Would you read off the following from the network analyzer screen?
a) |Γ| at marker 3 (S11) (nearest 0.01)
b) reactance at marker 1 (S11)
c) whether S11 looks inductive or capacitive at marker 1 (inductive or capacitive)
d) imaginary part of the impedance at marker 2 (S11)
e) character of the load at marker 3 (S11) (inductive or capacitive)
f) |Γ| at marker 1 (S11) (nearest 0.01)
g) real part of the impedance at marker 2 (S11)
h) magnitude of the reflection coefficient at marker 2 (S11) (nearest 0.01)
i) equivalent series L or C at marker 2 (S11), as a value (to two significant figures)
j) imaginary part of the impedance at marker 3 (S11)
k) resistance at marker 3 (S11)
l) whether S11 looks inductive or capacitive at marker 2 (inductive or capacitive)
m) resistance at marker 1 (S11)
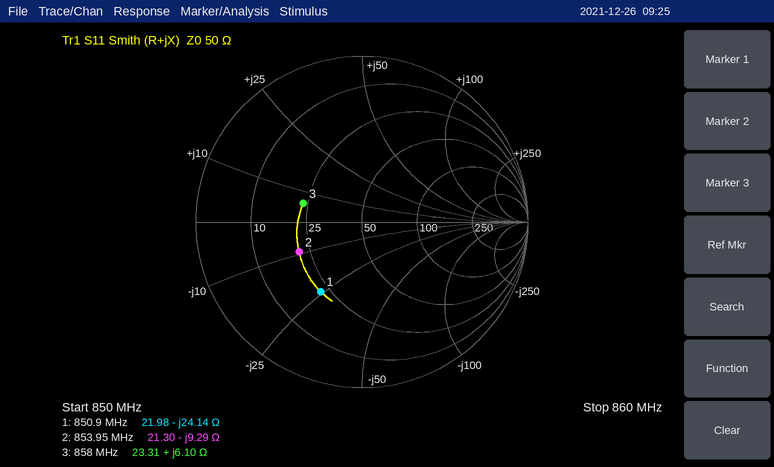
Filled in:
0.37
-24.14 Ω
capacitive
-9.29 Ω
inductive
0.49
21.30 Ω
0.42
20 pF
+6.10 Ω
23.31 Ω
capacitive
21.98 Ω
